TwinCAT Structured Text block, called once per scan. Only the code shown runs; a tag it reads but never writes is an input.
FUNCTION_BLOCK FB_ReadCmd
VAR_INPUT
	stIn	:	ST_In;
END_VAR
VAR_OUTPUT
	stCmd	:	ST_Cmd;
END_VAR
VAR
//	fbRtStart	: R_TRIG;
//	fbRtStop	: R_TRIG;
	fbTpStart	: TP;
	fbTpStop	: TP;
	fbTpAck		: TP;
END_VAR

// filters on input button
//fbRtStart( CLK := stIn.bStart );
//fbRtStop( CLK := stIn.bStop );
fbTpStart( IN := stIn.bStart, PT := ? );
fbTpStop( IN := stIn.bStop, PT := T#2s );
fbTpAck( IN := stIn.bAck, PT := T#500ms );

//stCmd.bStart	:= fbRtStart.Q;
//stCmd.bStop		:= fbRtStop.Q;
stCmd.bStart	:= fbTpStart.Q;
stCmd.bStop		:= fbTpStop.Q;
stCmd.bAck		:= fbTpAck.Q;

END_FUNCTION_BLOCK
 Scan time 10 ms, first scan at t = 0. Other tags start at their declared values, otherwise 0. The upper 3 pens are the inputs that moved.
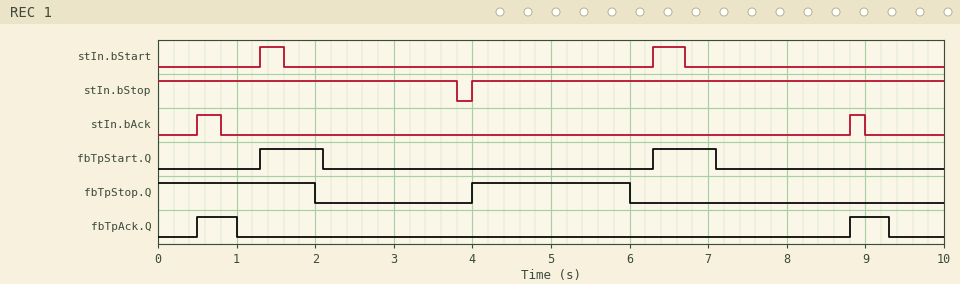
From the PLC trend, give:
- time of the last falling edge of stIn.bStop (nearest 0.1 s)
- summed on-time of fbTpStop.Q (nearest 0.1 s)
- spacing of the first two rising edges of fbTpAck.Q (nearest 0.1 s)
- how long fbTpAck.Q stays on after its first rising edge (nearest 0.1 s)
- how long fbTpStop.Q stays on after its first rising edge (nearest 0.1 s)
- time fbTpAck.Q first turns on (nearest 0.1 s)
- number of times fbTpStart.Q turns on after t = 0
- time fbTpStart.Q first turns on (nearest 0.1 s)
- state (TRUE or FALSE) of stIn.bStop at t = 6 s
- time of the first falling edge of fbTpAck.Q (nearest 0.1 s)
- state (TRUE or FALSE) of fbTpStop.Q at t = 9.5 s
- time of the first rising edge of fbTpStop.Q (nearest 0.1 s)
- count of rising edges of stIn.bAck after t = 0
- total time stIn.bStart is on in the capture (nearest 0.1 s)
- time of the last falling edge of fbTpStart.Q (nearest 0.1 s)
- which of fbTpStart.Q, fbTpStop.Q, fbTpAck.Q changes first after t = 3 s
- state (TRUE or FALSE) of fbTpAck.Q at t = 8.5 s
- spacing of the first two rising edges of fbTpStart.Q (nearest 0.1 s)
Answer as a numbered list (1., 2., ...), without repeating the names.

1. 3.8 s
2. 4.0 s
3. 8.3 s
4. 0.5 s
5. 2.0 s
6. 0.5 s
7. 2
8. 1.3 s
9. TRUE
10. 1.0 s
11. FALSE
12. 4.0 s
13. 2
14. 0.7 s
15. 7.1 s
16. fbTpStop.Q
17. FALSE
18. 5.0 s
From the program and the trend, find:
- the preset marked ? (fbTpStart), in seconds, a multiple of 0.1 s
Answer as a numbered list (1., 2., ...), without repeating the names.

1. 0.8 s
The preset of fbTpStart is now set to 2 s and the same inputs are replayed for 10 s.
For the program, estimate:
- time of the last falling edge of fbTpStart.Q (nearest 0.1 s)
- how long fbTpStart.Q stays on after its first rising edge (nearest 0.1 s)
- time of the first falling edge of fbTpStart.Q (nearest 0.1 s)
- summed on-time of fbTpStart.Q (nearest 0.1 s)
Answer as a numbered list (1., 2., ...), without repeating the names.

1. 8.3 s
2. 2.0 s
3. 3.3 s
4. 4.0 s
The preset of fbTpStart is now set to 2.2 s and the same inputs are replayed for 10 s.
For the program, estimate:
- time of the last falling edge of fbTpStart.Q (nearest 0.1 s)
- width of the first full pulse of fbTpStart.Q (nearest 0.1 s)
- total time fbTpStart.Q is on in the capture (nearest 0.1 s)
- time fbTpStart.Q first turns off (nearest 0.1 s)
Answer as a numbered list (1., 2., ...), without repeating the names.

1. 8.5 s
2. 2.2 s
3. 4.4 s
4. 3.5 s
